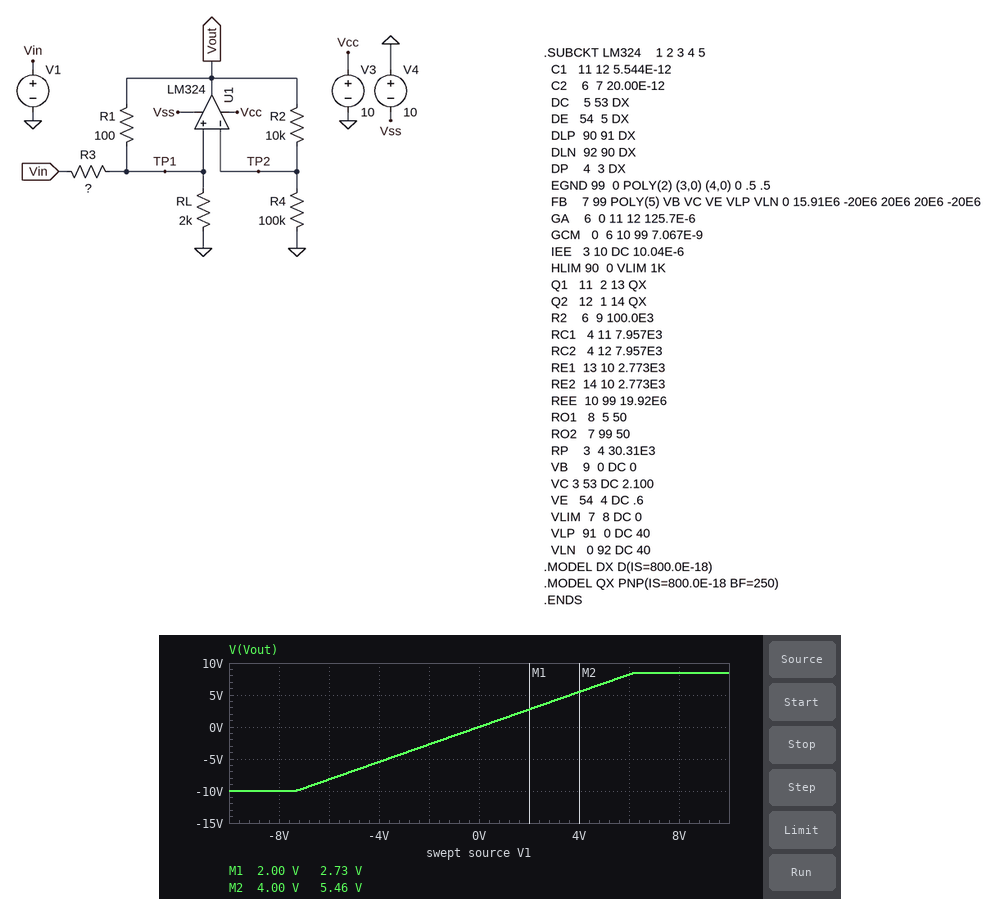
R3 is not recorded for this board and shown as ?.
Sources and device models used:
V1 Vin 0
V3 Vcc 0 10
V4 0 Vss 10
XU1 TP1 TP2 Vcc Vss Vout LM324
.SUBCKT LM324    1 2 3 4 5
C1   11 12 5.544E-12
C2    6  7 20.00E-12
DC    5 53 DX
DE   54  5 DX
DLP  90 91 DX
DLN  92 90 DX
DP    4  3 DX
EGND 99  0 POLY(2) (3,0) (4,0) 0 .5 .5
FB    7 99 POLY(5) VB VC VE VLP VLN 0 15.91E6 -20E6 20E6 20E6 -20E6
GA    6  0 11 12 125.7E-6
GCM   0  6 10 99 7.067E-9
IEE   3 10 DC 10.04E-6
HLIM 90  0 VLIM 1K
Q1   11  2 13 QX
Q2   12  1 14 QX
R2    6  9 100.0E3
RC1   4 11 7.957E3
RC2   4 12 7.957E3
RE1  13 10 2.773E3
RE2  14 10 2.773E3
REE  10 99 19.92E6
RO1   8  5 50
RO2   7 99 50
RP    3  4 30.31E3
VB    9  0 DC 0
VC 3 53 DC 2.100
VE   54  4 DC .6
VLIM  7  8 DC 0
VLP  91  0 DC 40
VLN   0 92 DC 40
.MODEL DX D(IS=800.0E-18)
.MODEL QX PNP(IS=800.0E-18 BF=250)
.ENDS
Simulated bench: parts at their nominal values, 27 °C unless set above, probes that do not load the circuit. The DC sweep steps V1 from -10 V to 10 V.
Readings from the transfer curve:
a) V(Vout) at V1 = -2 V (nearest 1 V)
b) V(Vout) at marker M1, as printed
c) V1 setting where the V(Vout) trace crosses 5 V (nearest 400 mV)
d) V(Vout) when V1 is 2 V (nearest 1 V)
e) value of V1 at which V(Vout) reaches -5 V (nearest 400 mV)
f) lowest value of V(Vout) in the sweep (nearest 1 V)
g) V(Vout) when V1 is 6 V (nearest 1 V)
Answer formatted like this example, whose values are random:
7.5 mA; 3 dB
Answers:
-3 V; 2.73 V; 3.6 V; 3 V; -3.6 V; -10 V; 8 V
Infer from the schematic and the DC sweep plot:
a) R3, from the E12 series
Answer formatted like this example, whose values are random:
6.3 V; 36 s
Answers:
390 Ω
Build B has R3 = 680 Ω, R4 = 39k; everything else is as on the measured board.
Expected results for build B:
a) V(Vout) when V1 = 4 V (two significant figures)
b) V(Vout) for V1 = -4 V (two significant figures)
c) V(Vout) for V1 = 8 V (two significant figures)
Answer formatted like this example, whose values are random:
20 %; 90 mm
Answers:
8.5 V; -10 V; 8.5 V
